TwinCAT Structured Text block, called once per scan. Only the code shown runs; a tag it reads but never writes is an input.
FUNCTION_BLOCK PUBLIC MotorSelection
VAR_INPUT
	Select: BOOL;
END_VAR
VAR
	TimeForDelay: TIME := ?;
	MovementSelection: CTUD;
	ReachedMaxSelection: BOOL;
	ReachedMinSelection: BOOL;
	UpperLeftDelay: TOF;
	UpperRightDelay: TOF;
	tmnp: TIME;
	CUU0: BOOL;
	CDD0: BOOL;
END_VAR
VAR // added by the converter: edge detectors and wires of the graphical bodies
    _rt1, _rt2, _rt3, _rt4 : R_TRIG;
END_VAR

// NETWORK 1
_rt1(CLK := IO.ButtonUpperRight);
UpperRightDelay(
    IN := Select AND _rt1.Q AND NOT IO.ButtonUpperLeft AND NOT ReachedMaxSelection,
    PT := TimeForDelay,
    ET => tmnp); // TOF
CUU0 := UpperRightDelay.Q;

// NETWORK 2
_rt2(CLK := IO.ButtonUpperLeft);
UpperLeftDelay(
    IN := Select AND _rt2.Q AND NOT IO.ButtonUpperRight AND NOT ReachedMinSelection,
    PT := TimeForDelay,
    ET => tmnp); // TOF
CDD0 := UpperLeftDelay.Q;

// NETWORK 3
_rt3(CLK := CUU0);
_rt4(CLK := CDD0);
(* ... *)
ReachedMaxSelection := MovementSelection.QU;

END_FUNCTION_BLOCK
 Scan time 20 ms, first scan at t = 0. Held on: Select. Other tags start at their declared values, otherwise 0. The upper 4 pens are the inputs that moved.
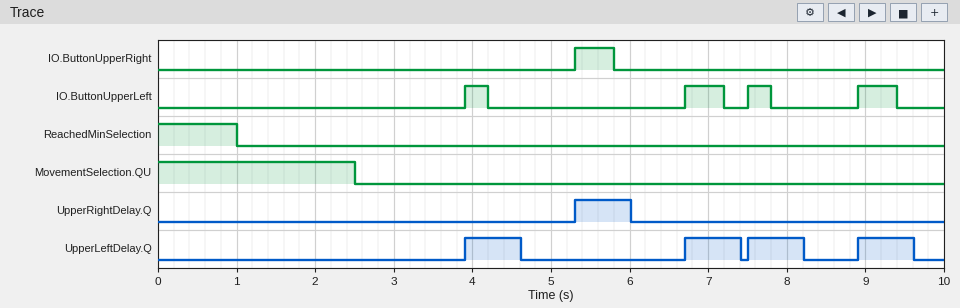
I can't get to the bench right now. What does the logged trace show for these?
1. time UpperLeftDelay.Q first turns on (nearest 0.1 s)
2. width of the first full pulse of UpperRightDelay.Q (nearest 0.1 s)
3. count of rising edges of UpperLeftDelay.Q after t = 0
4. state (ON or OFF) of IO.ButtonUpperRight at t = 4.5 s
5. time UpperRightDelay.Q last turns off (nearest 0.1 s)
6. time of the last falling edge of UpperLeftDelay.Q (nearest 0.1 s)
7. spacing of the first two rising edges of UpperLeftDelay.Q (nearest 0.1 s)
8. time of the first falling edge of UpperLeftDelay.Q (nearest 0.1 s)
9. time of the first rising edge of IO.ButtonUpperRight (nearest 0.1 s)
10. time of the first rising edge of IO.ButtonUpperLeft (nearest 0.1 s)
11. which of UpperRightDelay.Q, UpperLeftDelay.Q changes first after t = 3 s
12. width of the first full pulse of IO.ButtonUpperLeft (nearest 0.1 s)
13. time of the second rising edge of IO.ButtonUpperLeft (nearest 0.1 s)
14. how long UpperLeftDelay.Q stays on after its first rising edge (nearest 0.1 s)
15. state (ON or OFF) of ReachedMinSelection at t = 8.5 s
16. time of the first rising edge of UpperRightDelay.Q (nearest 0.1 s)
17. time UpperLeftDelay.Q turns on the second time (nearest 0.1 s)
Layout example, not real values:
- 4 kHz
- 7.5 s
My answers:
- 3.9 s
- 0.7 s
- 4
- OFF
- 6.0 s
- 9.6 s
- 2.8 s
- 4.6 s
- 5.3 s
- 3.9 s
- UpperLeftDelay.Q
- 0.3 s
- 6.7 s
- 0.7 s
- OFF
- 5.3 s
- 6.7 s
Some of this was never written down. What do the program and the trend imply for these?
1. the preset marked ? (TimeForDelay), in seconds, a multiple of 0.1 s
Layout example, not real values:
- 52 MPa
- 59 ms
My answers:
- 0.7 s
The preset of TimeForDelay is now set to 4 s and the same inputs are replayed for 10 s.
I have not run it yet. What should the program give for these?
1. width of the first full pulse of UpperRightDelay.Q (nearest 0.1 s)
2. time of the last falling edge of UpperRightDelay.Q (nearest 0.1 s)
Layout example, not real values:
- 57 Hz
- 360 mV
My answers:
- 4.0 s
- 9.3 s
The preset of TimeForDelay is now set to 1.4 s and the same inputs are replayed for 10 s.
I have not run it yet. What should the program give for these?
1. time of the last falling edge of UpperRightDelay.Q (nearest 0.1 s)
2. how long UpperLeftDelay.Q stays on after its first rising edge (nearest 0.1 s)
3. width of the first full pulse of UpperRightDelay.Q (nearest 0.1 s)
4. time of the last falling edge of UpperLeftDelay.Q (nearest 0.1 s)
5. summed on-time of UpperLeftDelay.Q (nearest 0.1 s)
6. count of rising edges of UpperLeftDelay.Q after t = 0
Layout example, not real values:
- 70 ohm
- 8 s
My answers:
- 6.7 s
- 1.4 s
- 1.4 s
- 5.3 s
- 4.7 s
- 2
